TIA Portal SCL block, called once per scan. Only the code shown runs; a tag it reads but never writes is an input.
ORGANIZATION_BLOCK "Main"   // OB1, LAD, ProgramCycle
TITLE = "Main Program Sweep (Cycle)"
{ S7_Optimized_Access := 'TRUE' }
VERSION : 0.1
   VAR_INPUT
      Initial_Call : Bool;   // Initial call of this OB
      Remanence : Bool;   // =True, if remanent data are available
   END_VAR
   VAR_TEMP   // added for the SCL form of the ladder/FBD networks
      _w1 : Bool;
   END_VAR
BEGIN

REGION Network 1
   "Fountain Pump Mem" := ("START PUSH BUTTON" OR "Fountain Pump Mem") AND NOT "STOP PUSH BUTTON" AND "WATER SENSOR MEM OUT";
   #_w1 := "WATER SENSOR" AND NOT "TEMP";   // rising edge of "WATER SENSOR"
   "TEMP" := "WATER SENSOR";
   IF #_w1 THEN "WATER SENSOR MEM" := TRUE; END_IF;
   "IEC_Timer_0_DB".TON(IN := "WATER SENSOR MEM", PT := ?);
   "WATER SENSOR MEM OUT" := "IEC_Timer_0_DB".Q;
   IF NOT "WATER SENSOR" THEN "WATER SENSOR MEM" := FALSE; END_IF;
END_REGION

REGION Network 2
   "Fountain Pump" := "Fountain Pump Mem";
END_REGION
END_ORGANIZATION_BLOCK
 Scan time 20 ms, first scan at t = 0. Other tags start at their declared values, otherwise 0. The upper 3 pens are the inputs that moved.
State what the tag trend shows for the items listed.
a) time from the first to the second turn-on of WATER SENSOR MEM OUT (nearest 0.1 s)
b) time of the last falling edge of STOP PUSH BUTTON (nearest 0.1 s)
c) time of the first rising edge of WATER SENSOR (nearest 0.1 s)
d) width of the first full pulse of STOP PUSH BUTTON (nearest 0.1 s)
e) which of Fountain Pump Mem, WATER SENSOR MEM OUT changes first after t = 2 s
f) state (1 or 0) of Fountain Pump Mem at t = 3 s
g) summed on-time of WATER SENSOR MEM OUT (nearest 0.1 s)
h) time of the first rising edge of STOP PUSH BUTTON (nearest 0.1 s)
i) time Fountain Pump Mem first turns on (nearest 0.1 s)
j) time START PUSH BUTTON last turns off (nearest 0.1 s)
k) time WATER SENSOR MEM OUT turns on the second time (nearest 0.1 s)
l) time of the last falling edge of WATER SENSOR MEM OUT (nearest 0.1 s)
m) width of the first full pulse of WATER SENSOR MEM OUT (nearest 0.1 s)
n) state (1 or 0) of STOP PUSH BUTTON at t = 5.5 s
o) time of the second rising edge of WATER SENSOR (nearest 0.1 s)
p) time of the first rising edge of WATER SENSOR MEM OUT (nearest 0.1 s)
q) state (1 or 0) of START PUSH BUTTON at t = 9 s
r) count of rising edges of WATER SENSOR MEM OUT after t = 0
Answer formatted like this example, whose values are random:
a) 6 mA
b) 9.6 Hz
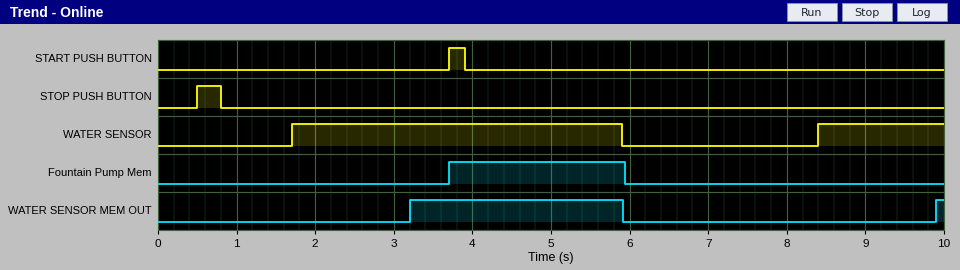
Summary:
a) 6.7 s
b) 0.8 s
c) 1.7 s
d) 0.3 s
e) WATER SENSOR MEM OUT
f) 0
g) 2.8 s
h) 0.5 s
i) 3.7 s
j) 3.9 s
k) 9.9 s
l) 5.9 s
m) 2.7 s
n) 0
o) 8.4 s
p) 3.2 s
q) 0
r) 2
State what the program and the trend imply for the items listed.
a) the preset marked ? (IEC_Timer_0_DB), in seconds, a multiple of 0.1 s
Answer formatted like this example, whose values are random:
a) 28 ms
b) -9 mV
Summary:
a) 1.5 s
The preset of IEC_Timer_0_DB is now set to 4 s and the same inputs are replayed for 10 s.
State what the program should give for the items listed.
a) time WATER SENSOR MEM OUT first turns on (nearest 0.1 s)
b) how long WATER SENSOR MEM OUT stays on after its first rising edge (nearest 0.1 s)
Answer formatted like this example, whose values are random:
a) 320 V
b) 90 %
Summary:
a) 5.7 s
b) 0.2 s
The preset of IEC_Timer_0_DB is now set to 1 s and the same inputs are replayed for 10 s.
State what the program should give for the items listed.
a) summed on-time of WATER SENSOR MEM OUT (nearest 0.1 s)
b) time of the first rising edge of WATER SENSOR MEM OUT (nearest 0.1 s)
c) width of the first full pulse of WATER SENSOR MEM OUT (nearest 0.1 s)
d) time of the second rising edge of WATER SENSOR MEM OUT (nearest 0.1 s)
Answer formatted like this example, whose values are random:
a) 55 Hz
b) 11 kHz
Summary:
a) 3.8 s
b) 2.7 s
c) 3.2 s
d) 9.4 s
